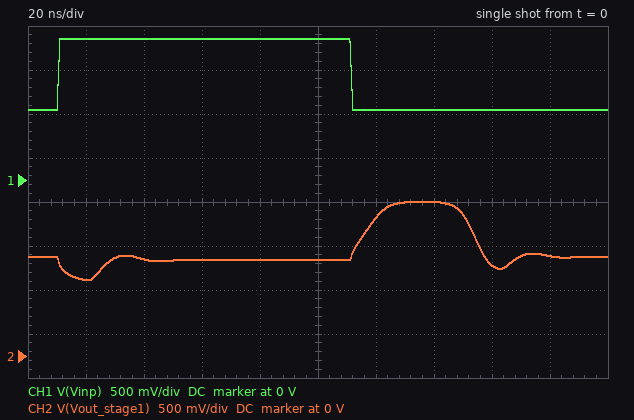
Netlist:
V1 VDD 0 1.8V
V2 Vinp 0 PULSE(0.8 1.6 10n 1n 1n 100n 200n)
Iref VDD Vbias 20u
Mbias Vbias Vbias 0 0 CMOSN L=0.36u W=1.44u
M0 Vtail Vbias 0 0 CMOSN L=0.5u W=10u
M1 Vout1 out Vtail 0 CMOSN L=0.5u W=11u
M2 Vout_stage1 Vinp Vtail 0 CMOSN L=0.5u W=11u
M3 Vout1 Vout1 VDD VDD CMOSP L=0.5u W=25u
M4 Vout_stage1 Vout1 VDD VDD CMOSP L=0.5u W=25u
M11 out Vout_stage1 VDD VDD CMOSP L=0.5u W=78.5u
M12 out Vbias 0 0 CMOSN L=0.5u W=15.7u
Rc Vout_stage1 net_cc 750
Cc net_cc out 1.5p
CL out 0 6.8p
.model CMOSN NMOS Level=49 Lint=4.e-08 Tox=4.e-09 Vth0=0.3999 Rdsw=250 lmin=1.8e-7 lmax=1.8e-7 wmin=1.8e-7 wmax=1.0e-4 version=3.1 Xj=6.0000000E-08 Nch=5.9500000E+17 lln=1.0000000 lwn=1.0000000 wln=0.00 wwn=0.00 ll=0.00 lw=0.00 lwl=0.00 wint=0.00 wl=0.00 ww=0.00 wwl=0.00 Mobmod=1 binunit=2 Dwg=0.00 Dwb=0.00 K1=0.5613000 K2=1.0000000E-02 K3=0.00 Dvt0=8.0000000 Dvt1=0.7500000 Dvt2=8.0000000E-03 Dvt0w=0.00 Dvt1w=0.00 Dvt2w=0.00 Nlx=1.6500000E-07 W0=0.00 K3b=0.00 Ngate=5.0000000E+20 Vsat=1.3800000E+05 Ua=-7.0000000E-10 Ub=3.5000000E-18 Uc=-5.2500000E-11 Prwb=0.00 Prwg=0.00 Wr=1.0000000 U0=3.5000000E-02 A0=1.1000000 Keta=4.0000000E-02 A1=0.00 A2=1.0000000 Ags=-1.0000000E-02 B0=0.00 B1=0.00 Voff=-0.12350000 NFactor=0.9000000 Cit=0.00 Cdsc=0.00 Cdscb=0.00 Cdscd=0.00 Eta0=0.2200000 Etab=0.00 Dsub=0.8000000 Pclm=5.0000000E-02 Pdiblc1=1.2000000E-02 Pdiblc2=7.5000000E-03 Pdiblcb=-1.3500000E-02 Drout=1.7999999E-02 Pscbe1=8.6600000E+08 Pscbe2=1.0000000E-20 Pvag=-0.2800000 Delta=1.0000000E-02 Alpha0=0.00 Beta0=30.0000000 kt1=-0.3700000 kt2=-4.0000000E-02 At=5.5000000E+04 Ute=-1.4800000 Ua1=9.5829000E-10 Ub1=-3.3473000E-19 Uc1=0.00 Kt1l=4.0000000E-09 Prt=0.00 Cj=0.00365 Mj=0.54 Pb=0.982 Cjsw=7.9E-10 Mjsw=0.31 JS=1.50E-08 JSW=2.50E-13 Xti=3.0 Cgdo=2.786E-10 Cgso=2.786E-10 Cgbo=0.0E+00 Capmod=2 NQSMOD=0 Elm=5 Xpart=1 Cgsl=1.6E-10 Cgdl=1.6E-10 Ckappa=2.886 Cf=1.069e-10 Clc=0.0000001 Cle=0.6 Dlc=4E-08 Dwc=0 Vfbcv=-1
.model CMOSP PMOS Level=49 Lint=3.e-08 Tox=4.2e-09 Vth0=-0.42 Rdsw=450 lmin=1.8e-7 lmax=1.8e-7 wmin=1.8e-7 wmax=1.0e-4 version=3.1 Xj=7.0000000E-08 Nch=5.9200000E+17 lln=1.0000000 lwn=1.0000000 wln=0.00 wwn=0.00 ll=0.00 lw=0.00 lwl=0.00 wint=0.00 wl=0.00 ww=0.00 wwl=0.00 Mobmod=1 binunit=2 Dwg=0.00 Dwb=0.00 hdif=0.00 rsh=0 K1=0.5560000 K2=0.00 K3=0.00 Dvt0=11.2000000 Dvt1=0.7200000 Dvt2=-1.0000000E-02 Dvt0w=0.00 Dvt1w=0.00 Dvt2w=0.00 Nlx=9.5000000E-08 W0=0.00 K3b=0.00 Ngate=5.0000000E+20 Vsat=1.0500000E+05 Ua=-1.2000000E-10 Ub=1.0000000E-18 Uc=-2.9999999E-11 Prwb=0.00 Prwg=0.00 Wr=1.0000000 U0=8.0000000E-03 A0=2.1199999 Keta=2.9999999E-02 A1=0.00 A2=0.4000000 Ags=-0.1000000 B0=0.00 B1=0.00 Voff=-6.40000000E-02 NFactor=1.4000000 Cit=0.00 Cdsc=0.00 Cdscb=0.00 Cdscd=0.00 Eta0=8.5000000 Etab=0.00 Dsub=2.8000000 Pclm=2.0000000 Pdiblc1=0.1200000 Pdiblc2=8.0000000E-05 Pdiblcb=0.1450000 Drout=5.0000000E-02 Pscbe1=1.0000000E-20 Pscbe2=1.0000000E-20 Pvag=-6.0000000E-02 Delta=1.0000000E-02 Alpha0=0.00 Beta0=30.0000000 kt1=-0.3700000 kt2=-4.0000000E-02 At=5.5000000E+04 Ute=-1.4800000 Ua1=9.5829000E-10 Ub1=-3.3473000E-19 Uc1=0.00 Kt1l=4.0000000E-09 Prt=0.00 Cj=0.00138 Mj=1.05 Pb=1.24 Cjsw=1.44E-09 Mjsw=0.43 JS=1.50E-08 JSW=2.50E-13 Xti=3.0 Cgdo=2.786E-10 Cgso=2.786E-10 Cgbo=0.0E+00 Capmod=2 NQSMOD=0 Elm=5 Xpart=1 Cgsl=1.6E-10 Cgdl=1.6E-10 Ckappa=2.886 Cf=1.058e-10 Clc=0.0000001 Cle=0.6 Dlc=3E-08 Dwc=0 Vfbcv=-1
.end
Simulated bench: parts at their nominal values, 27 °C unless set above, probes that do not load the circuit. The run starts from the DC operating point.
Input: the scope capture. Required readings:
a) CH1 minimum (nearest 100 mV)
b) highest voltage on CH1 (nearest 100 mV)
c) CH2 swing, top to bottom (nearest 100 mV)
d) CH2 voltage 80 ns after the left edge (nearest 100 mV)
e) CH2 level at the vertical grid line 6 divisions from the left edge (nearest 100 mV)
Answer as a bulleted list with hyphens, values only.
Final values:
- 800 mV
- 1.6 V
- 900 mV
- 1.1 V
- 1.6 V
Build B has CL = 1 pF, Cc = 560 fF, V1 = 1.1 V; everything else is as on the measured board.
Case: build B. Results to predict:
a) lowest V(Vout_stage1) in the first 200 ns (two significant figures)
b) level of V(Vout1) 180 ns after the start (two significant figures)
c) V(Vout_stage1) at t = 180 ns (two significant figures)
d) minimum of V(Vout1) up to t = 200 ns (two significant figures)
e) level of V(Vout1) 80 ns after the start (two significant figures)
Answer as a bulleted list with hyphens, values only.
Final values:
- 300 mV
- 440 mV
- 410 mV
- 360 mV
- 430 mV
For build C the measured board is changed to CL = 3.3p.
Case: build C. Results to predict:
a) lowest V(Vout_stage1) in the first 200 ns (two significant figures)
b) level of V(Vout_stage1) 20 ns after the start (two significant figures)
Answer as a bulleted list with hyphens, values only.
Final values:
- 940 mV
- 950 mV
